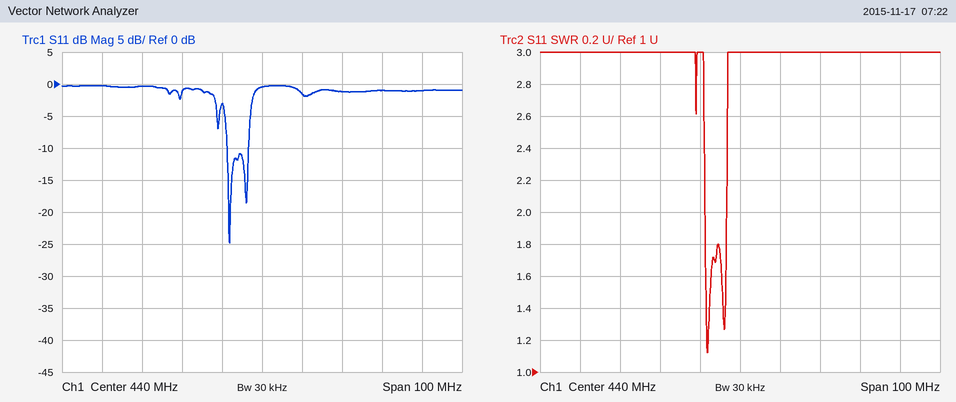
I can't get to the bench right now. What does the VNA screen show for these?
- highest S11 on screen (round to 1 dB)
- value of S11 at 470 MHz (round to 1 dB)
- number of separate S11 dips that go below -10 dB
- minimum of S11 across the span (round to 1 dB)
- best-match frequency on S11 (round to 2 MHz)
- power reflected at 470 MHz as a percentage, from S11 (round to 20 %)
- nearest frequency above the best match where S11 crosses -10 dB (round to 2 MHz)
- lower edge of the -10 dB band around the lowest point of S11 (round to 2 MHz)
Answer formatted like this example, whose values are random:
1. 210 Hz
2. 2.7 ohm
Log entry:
1. 0 dB
2. -1 dB
3. 2
4. -25 dB
5. 432 MHz
6. 80 %
7. 436 MHz
8. 432 MHz
